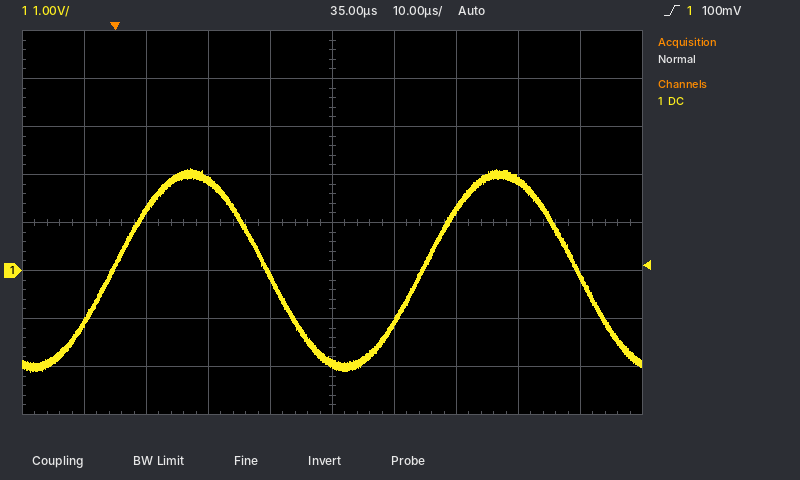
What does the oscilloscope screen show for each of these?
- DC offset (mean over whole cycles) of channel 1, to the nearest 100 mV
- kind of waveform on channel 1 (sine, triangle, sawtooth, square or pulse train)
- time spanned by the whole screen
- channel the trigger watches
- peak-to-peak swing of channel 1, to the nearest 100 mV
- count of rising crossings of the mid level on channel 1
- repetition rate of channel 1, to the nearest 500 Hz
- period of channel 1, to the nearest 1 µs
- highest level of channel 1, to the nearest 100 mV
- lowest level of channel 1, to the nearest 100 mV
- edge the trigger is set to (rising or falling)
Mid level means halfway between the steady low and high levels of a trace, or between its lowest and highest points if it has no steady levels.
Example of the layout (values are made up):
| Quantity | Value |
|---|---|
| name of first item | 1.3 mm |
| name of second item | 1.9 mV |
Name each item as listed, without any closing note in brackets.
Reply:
| Quantity | Value |
|---|---|
| DC offset (mean over whole cycles) of channel 1, to the nearest 100 mV | 0.0 V |
| kind of waveform on channel 1 | sine |
| time spanned by the whole screen | 100 µs |
| channel the trigger watches | channel 1 |
| peak-to-peak swing of channel 1, to the nearest 100 mV | 4.2 V |
| count of rising crossings of the mid level on channel 1 | 2 |
| repetition rate of channel 1, to the nearest 500 Hz | 20.0 kHz |
| period of channel 1, to the nearest 1 µs | 50 µs |
| highest level of channel 1, to the nearest 100 mV | 2.1 V |
| lowest level of channel 1, to the nearest 100 mV | -2.1 V |
| edge the trigger is set to | rising |
